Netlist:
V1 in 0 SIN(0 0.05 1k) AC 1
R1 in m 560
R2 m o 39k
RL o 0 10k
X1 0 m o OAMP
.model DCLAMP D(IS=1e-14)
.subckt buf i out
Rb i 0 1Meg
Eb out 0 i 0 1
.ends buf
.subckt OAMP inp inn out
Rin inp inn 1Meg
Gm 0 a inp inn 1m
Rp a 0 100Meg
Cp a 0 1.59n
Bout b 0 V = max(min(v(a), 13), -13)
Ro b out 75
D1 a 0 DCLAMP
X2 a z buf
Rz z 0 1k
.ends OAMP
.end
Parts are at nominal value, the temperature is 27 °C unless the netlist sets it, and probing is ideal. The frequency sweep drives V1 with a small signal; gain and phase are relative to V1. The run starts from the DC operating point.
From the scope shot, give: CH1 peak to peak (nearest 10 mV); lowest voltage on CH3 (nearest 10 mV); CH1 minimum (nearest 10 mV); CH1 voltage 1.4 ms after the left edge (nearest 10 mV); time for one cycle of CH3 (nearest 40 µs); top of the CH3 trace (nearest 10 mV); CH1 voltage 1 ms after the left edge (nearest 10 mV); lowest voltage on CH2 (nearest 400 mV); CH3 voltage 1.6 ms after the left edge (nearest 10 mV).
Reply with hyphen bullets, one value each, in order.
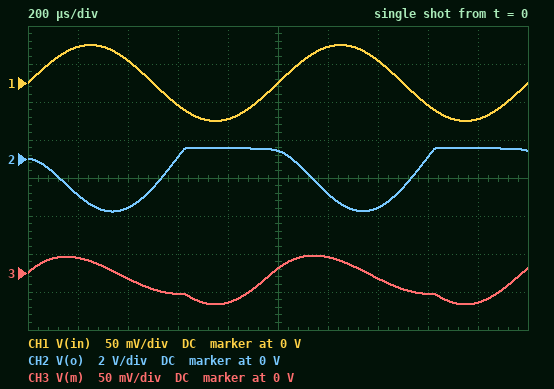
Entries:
- 100 mV
- -40 mV
- -50 mV
- 30 mV
- 1.00 ms
- 20 mV
- 0 V
- -2.8 V
- -30 mV
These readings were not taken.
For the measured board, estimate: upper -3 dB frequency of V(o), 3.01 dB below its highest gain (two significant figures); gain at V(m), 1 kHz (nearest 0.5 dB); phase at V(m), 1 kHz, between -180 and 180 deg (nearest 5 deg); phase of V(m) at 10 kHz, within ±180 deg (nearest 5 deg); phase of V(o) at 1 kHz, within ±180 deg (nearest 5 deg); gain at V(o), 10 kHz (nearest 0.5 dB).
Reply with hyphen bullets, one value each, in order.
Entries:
- 1.5 kHz
- -5.0 dB
- 50 deg
- 10 deg
- 145 deg
- 19.5 dB
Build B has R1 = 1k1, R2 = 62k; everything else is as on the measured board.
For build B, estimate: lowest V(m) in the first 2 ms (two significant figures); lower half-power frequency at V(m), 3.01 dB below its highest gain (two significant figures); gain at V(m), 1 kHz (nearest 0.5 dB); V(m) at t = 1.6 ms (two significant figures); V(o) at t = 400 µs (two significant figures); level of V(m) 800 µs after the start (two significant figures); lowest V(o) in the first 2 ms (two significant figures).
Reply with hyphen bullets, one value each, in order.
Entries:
- -39 mV
- 1.8 kHz
- -6.5 dB
- -24 mV
- -2.1 V
- -37 mV
- -2.4 V
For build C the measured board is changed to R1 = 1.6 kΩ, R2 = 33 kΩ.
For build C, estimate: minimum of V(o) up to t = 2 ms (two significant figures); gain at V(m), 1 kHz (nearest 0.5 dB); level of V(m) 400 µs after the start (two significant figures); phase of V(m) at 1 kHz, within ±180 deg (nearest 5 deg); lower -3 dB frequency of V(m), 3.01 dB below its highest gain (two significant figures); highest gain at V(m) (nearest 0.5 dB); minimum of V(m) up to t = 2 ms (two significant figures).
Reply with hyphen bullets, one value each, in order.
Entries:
- -990 mV
- -14.0 dB
- -5.9 mV
- 70 deg
- 4.7 kHz
- -0.5 dB
- -22 mV
